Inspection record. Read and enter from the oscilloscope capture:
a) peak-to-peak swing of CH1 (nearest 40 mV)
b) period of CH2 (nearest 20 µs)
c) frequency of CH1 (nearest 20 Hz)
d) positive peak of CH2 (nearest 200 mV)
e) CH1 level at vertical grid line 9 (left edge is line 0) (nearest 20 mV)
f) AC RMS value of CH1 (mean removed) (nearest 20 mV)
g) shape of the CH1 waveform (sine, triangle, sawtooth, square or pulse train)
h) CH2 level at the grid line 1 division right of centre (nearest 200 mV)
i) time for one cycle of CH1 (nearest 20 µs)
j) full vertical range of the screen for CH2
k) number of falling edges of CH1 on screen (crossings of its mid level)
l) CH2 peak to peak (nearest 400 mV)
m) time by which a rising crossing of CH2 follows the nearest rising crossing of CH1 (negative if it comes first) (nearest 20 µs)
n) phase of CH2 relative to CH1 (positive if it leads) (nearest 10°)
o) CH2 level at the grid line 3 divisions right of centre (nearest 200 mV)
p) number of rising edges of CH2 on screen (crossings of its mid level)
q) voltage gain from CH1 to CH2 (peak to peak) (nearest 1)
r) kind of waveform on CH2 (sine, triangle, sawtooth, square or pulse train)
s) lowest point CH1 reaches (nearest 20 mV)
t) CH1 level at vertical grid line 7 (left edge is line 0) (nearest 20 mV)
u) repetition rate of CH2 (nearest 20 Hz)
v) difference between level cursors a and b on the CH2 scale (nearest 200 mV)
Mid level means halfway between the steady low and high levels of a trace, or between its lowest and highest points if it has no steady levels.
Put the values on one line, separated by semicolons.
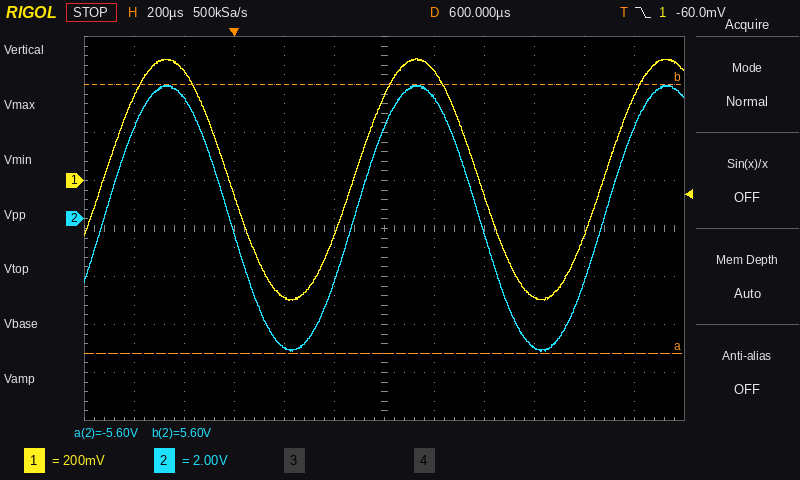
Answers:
1.00 V; 1.00 ms; 1.00 kHz; 5.6 V; -480 mV; 360 mV; sine; 5.0 V; 1.00 ms; 16 V; 2; 11.2 V; 0 µs; 0°; -5.4 V; 3; 11; sine; -500 mV; 460 mV; 1.00 kHz; 11.2 V
